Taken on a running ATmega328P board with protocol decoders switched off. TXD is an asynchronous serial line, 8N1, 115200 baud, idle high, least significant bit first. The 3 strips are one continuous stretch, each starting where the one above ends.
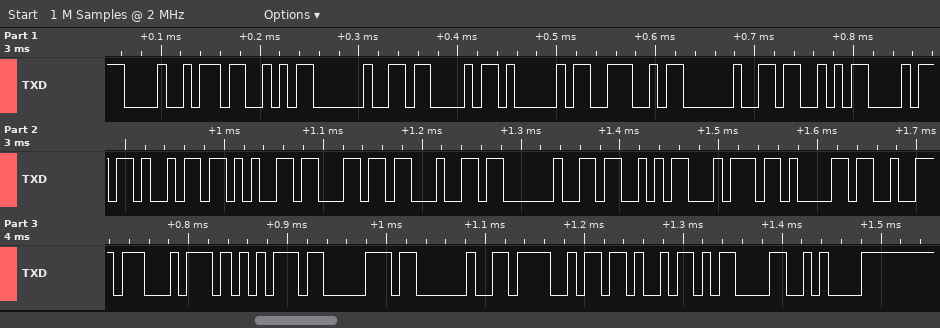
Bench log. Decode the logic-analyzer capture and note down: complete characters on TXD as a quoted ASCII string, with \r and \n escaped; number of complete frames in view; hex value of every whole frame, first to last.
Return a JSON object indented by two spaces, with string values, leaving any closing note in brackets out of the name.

{
  "complete characters on TXD as a quoted ASCII string, with \\r and \\n escaped": "\"HS CAN Shield Startup OK\\r\\n\"",
  "number of complete frames in view": "26",
  "hex value of every whole frame, first to last": "48 53 20 43 41 4E 20 53 68 69 65 6C 64 20 53 74 61 72 74 75 70 20 4F 4B 0D 0A"
}
